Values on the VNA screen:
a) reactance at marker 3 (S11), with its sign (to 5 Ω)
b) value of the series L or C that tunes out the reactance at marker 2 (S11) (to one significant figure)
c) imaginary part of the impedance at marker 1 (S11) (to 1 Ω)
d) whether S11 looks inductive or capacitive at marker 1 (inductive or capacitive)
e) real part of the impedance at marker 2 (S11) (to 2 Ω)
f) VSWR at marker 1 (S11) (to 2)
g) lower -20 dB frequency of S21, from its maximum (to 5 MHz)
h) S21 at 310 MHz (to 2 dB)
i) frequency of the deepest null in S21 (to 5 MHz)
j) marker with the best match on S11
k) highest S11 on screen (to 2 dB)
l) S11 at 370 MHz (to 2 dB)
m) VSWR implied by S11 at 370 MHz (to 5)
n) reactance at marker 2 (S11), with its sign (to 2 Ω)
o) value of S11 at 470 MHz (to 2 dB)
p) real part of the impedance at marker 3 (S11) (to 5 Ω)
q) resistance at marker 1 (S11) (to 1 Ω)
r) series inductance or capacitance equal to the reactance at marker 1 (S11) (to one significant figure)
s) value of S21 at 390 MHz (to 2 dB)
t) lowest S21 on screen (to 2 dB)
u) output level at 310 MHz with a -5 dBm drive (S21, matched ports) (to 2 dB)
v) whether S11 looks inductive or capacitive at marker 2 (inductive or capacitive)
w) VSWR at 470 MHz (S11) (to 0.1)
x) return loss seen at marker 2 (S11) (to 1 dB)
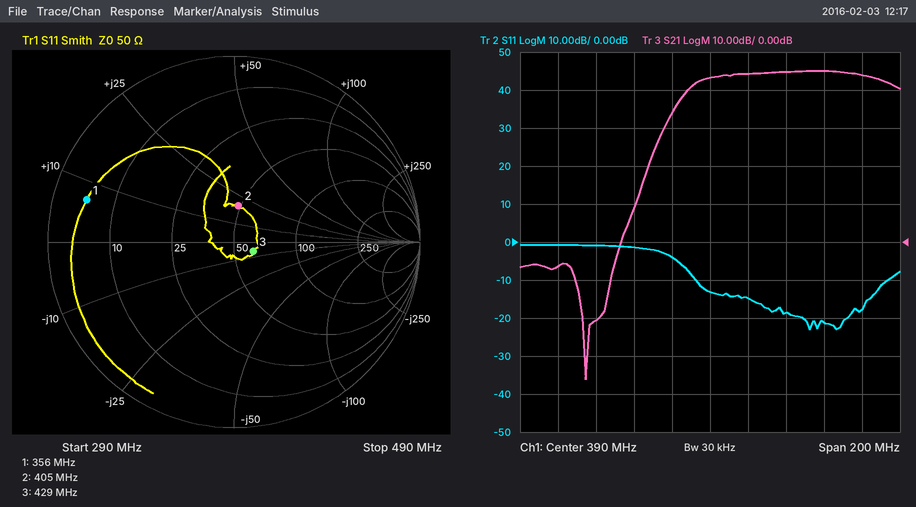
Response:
-5 Ω
20 pF
+7 Ω
inductive
48 Ω
10
360 MHz
-6 dB
325 MHz
marker 3
0 dB
-4 dB
5
+20 Ω
-18 dB
60 Ω
5 Ω
3 nH
44 dB
-36 dB
-12 dBm
inductive
1.3
14 dB
